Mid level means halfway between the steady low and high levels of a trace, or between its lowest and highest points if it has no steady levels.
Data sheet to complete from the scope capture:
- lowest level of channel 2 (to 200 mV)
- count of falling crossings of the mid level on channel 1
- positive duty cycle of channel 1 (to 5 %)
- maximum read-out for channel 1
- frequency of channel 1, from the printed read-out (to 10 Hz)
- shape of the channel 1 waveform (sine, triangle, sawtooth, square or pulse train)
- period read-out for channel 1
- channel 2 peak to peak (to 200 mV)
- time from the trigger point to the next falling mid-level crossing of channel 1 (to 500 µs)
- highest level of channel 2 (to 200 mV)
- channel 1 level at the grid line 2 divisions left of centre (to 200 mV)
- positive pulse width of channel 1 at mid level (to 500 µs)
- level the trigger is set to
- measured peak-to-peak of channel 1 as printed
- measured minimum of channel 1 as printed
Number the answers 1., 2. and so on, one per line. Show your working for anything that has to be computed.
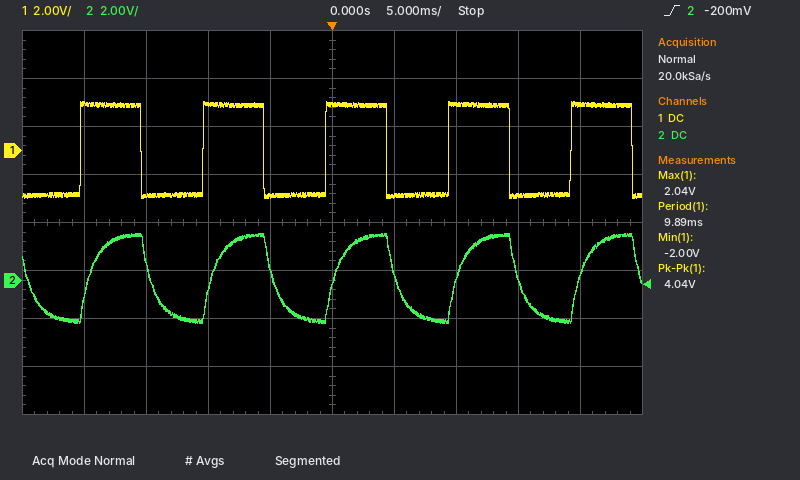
1. -1.8 V
2. 5
3. 50 %
4. 2.04 V
5. 1 / 9.89 ms ≈ 101 Hz, so 100 Hz to the nearest 10 Hz
6. square
7. 9.89 ms
8. 2.0 V − (-1.8 V) = 3.8 V
9. 4.5 ms
10. 2.0 V
11. 2.0 V
12. 5.0 ms
13. -200 mV
14. 4.04 V
15. -2.00 V
